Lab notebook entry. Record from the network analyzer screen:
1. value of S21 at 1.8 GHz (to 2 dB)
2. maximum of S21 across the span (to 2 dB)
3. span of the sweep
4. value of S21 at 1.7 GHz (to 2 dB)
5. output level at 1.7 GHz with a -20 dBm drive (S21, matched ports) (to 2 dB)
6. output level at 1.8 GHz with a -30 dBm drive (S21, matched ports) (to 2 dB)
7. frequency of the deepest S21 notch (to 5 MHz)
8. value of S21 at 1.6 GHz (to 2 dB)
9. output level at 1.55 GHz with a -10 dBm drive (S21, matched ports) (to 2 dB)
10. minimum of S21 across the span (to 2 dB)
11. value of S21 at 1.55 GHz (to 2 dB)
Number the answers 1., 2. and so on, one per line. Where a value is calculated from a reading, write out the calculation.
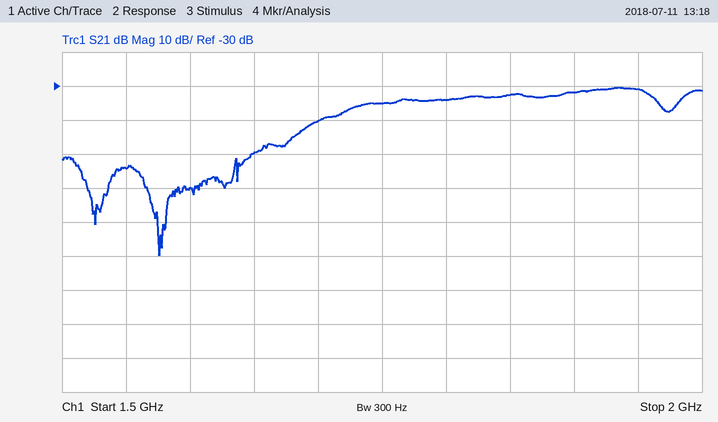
1. -34 dB
2. -30 dB
3. 500 MHz
4. -40 dB
5. -20 dBm + (-40 dB) = -60 dBm
6. -30 dBm + (-34 dB) = -64 dBm
7. 1.575 GHz
8. -60 dB
9. -10 dBm + (-54 dB) = -64 dBm
10. -80 dB
11. -54 dB
